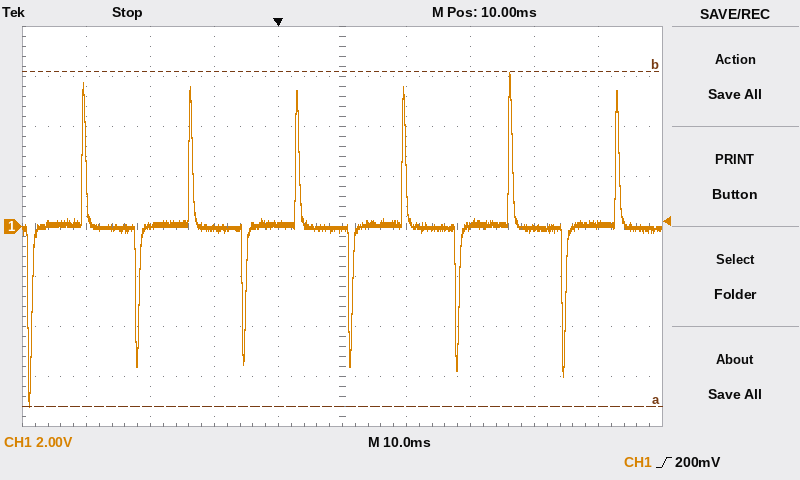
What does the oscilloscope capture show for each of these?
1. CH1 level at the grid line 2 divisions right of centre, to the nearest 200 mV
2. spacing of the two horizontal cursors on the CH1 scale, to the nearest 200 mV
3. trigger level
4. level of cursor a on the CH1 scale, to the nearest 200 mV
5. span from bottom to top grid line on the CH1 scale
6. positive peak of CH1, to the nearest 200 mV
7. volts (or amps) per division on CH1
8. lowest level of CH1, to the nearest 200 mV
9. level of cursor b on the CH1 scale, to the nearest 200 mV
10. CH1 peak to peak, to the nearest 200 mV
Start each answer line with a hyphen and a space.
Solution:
- 0.0 V
- 13.4 V
- 200 mV
- -7.2 V
- 16 V
- 6.2 V
- 2 V
- -7.2 V
- 6.2 V
- 13.4 V
